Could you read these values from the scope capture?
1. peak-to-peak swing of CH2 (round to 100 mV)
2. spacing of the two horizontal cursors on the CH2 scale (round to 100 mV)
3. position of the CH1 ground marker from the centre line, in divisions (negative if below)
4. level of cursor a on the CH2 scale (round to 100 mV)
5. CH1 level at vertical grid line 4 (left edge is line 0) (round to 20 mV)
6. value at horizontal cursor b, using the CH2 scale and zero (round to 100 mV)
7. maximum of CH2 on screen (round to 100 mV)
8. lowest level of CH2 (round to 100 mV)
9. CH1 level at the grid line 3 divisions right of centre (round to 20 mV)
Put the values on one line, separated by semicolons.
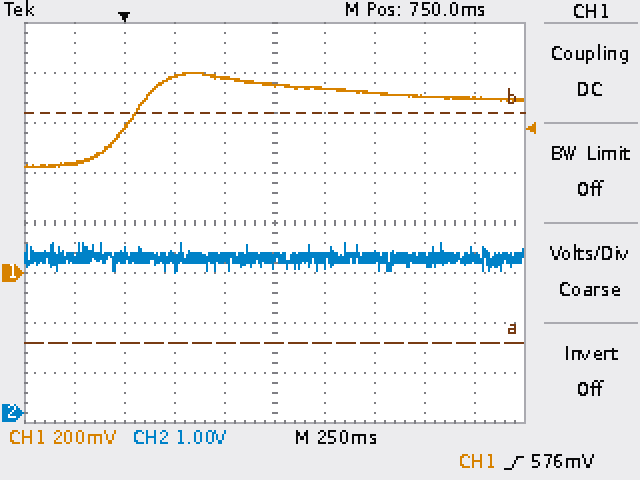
600 mV; 4.6 V; -1.0 div; 1.4 V; 780 mV; 6.0 V; 3.4 V; 2.8 V; 700 mV
